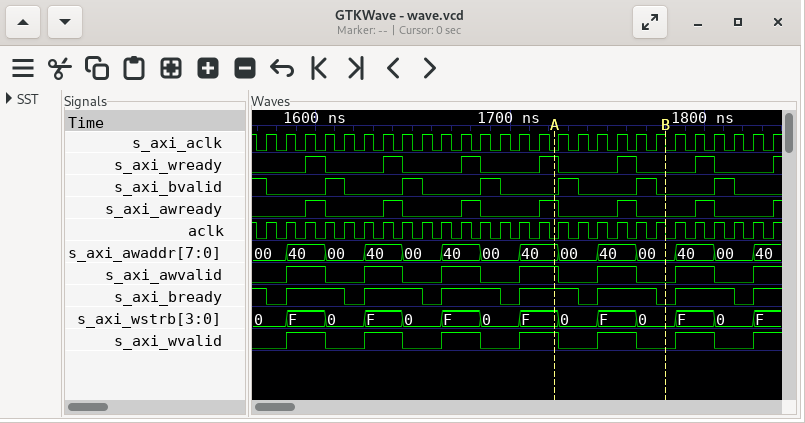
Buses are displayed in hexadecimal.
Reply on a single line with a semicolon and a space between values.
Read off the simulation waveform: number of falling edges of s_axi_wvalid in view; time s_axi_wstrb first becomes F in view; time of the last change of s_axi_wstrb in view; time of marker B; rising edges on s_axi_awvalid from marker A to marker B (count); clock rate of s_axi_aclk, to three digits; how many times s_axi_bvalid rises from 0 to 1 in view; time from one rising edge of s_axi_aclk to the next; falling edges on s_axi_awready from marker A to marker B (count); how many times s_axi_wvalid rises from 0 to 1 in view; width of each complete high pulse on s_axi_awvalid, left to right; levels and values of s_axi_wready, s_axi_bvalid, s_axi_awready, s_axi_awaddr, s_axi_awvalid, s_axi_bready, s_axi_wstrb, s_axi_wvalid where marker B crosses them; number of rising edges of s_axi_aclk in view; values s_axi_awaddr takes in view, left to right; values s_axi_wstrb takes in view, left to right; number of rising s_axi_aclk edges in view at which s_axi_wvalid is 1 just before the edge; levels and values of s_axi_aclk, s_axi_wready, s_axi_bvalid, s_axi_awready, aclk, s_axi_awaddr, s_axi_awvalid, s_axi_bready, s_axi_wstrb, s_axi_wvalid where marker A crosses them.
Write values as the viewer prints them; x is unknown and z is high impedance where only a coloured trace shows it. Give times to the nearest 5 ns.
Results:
6; 1585 ns; 1825 ns; 1780 ns; 1; 100 MHz; 6; 10 ns; 2; 7; 20 ns, 20 ns, 20 ns, 20 ns, 20 ns, 20 ns; s_axi_wready=0, s_axi_bvalid=0, s_axi_awready=0, s_axi_awaddr=00, s_axi_awvalid=0, s_axi_bready=0, s_axi_wstrb=0, s_axi_wvalid=0; 27; 00, 40, 00, 40, 00, 40, 00, 40, 00, 40, 00, 40, 00, 40; 0, F, 0, F, 0, F, 0, F, 0, F, 0, F, 0, F; 13; s_axi_aclk=0, s_axi_wready=1, s_axi_bvalid=0, s_axi_awready=1, aclk=0, s_axi_awaddr=40, s_axi_awvalid=1, s_axi_bready=1, s_axi_wstrb=F, s_axi_wvalid=1
